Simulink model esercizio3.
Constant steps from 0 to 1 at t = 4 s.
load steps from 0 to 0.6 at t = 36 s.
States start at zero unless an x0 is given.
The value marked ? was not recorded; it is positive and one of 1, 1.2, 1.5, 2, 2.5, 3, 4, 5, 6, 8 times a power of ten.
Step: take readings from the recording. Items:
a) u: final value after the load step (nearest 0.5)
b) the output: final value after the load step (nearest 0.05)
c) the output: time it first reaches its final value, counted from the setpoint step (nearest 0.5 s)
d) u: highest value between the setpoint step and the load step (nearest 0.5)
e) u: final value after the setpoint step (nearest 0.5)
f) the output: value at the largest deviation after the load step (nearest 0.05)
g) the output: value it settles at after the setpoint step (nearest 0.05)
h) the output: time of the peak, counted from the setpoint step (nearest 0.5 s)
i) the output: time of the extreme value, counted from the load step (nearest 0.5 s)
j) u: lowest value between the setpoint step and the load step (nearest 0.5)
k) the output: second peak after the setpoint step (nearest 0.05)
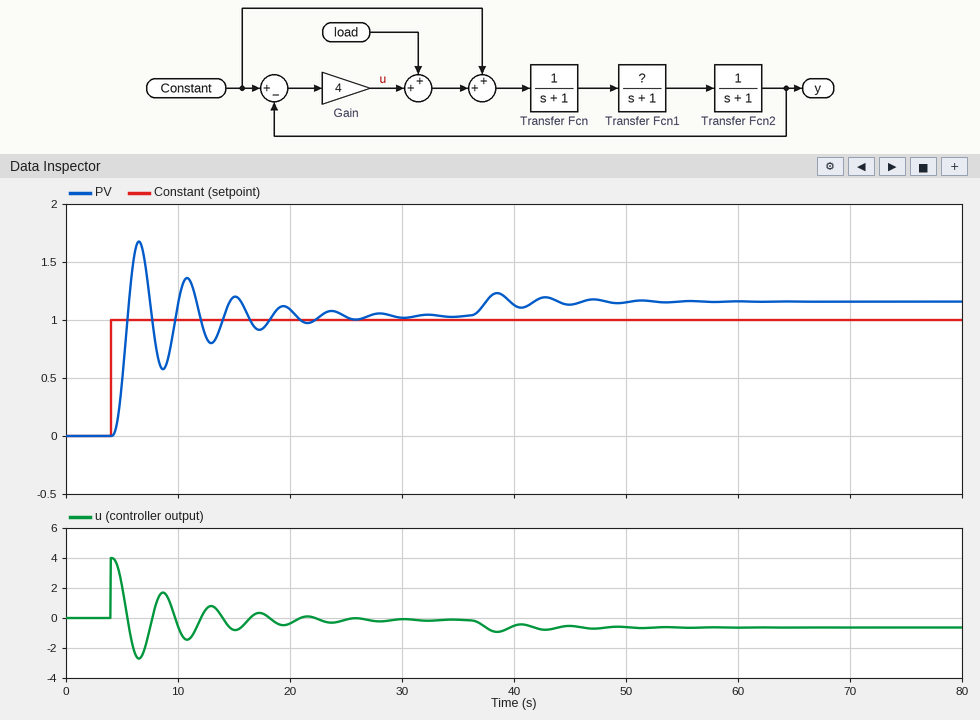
-0.5
1.15
1.5 s
4.0
0.0
1.25
1.05
2.5 s
2.5 s
-2.5
1.35
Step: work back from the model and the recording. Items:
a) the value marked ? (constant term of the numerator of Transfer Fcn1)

1.2
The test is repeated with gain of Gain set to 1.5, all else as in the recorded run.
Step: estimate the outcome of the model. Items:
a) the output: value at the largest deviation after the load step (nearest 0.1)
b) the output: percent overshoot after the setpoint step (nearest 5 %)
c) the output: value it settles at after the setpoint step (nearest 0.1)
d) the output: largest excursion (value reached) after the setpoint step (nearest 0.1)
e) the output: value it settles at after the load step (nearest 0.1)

1.4
25 %
1.1
1.4
1.3
